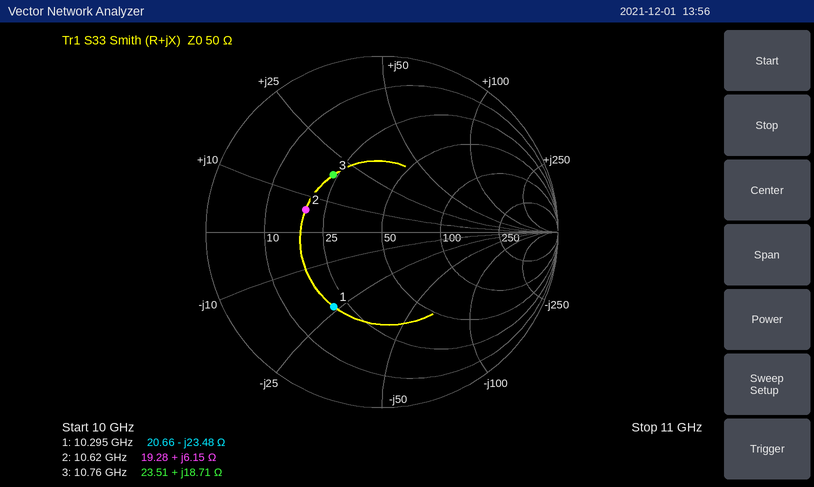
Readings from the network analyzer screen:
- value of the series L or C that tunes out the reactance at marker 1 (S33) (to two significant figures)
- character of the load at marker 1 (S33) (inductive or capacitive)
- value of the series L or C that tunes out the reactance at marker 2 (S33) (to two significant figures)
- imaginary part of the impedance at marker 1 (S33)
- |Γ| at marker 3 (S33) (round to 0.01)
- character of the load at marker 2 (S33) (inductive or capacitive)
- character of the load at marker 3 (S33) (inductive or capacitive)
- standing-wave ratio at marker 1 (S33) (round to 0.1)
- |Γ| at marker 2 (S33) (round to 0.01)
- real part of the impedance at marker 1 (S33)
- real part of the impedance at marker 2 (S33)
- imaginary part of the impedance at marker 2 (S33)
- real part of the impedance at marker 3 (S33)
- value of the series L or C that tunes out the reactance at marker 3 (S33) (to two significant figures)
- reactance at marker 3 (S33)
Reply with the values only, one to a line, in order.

360 pH
capacitive
2.4 pF
-23.48 Ω
0.43
inductive
inductive
3.0
0.45
20.66 Ω
19.28 Ω
+6.15 Ω
23.51 Ω
790 fF
+18.71 Ω
